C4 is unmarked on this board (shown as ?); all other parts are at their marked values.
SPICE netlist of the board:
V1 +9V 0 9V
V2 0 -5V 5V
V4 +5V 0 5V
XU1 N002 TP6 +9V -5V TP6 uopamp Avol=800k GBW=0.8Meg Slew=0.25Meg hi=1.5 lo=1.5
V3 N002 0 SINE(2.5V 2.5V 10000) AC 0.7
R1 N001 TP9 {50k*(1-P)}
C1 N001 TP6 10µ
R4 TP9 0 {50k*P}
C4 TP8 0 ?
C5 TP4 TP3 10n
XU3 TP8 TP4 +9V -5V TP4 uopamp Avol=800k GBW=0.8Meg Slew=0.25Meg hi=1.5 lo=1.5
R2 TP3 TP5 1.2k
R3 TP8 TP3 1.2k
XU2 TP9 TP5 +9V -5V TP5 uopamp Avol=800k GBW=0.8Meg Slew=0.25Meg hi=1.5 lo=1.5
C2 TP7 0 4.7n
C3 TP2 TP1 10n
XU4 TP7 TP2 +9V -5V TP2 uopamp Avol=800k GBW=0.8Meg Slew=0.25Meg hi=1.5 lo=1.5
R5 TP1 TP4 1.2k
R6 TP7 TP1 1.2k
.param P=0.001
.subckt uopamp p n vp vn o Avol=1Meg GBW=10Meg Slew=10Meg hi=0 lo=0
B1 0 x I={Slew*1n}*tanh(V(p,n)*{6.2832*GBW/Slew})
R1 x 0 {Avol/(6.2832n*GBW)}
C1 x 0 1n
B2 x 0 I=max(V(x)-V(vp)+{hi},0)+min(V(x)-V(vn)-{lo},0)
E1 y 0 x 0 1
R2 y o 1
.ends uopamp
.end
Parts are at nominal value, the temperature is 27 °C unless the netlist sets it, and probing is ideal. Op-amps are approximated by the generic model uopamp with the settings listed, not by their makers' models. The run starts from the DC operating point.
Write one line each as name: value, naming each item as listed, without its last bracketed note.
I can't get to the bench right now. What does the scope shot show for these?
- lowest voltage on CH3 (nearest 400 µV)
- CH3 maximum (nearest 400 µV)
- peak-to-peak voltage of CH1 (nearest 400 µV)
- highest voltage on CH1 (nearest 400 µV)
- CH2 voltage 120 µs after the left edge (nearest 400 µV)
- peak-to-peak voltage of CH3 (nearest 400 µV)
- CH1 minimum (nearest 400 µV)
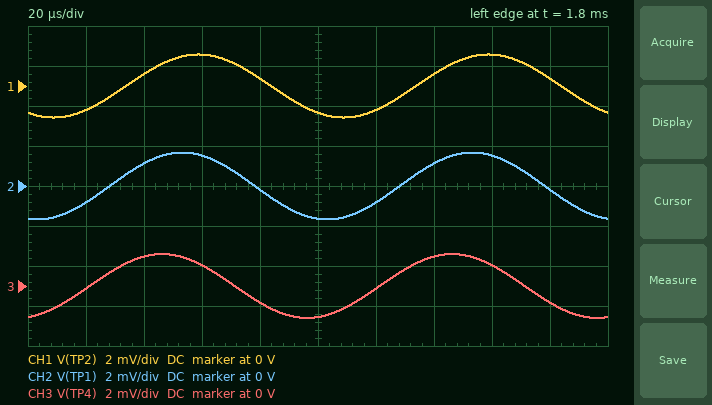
lowest voltage on CH3: -1.6 mV
CH3 maximum: 1.6 mV
peak-to-peak voltage of CH1: 3.2 mV
highest voltage on CH1: 1.6 mV
CH2 voltage 120 µs after the left edge: -800 µV
peak-to-peak voltage of CH3: 3.2 mV
CH1 minimum: -1.6 mV
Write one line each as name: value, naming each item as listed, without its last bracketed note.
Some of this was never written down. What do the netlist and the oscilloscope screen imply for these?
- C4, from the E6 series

C4, from the E6 series: 10 nF
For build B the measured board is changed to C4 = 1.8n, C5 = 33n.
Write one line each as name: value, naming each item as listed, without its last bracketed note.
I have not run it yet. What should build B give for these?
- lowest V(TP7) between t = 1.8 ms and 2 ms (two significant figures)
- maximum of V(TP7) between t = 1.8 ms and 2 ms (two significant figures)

lowest V(TP7) between t = 1.8 ms and 2 ms: -3.6 mV
maximum of V(TP7) between t = 1.8 ms and 2 ms: 3.6 mV
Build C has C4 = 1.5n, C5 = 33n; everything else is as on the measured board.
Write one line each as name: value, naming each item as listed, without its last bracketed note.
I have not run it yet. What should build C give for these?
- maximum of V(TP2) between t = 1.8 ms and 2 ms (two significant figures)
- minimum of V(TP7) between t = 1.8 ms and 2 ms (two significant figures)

maximum of V(TP2) between t = 1.8 ms and 2 ms: 3.4 mV
minimum of V(TP7) between t = 1.8 ms and 2 ms: -3.4 mV
